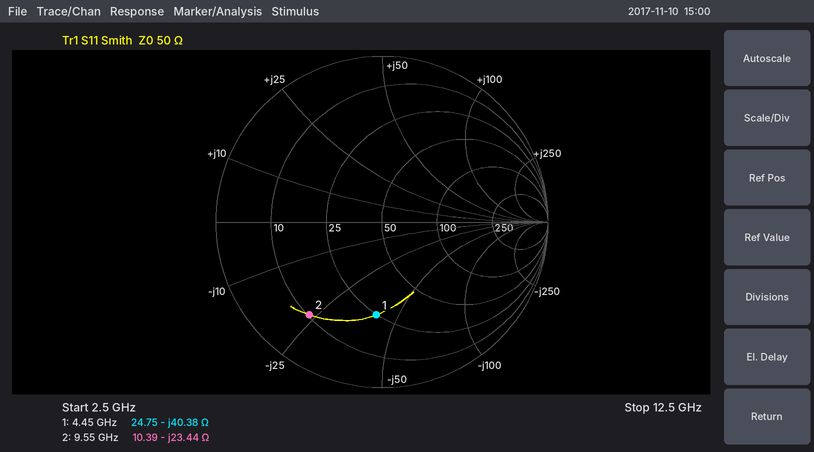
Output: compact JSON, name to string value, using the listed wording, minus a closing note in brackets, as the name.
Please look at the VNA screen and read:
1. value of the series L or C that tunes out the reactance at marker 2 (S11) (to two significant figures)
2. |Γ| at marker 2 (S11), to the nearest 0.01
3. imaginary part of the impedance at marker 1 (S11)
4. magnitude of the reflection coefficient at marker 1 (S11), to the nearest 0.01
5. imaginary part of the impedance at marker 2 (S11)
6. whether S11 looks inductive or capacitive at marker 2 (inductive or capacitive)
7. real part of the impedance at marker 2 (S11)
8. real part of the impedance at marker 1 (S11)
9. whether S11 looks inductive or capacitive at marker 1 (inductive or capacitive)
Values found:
{"value of the series L or C that tunes out the reactance at marker 2 (S11)": "390 pH", "|Γ| at marker 2 (S11), to the nearest 0.01": "0.71", "imaginary part of the impedance at marker 1": "-40.38 Ω", "magnitude of the reflection coefficient at marker 1 (S11), to the nearest 0.01": "0.56", "imaginary part of the impedance at marker 2": "-23.44 Ω", "whether S11 looks inductive or capacitive at marker 2": "capacitive", "real part of the impedance at marker 2": "10.39 Ω", "real part of the impedance at marker 1": "24.75 Ω", "whether S11 looks inductive or capacitive at marker 1": "capacitive"}
